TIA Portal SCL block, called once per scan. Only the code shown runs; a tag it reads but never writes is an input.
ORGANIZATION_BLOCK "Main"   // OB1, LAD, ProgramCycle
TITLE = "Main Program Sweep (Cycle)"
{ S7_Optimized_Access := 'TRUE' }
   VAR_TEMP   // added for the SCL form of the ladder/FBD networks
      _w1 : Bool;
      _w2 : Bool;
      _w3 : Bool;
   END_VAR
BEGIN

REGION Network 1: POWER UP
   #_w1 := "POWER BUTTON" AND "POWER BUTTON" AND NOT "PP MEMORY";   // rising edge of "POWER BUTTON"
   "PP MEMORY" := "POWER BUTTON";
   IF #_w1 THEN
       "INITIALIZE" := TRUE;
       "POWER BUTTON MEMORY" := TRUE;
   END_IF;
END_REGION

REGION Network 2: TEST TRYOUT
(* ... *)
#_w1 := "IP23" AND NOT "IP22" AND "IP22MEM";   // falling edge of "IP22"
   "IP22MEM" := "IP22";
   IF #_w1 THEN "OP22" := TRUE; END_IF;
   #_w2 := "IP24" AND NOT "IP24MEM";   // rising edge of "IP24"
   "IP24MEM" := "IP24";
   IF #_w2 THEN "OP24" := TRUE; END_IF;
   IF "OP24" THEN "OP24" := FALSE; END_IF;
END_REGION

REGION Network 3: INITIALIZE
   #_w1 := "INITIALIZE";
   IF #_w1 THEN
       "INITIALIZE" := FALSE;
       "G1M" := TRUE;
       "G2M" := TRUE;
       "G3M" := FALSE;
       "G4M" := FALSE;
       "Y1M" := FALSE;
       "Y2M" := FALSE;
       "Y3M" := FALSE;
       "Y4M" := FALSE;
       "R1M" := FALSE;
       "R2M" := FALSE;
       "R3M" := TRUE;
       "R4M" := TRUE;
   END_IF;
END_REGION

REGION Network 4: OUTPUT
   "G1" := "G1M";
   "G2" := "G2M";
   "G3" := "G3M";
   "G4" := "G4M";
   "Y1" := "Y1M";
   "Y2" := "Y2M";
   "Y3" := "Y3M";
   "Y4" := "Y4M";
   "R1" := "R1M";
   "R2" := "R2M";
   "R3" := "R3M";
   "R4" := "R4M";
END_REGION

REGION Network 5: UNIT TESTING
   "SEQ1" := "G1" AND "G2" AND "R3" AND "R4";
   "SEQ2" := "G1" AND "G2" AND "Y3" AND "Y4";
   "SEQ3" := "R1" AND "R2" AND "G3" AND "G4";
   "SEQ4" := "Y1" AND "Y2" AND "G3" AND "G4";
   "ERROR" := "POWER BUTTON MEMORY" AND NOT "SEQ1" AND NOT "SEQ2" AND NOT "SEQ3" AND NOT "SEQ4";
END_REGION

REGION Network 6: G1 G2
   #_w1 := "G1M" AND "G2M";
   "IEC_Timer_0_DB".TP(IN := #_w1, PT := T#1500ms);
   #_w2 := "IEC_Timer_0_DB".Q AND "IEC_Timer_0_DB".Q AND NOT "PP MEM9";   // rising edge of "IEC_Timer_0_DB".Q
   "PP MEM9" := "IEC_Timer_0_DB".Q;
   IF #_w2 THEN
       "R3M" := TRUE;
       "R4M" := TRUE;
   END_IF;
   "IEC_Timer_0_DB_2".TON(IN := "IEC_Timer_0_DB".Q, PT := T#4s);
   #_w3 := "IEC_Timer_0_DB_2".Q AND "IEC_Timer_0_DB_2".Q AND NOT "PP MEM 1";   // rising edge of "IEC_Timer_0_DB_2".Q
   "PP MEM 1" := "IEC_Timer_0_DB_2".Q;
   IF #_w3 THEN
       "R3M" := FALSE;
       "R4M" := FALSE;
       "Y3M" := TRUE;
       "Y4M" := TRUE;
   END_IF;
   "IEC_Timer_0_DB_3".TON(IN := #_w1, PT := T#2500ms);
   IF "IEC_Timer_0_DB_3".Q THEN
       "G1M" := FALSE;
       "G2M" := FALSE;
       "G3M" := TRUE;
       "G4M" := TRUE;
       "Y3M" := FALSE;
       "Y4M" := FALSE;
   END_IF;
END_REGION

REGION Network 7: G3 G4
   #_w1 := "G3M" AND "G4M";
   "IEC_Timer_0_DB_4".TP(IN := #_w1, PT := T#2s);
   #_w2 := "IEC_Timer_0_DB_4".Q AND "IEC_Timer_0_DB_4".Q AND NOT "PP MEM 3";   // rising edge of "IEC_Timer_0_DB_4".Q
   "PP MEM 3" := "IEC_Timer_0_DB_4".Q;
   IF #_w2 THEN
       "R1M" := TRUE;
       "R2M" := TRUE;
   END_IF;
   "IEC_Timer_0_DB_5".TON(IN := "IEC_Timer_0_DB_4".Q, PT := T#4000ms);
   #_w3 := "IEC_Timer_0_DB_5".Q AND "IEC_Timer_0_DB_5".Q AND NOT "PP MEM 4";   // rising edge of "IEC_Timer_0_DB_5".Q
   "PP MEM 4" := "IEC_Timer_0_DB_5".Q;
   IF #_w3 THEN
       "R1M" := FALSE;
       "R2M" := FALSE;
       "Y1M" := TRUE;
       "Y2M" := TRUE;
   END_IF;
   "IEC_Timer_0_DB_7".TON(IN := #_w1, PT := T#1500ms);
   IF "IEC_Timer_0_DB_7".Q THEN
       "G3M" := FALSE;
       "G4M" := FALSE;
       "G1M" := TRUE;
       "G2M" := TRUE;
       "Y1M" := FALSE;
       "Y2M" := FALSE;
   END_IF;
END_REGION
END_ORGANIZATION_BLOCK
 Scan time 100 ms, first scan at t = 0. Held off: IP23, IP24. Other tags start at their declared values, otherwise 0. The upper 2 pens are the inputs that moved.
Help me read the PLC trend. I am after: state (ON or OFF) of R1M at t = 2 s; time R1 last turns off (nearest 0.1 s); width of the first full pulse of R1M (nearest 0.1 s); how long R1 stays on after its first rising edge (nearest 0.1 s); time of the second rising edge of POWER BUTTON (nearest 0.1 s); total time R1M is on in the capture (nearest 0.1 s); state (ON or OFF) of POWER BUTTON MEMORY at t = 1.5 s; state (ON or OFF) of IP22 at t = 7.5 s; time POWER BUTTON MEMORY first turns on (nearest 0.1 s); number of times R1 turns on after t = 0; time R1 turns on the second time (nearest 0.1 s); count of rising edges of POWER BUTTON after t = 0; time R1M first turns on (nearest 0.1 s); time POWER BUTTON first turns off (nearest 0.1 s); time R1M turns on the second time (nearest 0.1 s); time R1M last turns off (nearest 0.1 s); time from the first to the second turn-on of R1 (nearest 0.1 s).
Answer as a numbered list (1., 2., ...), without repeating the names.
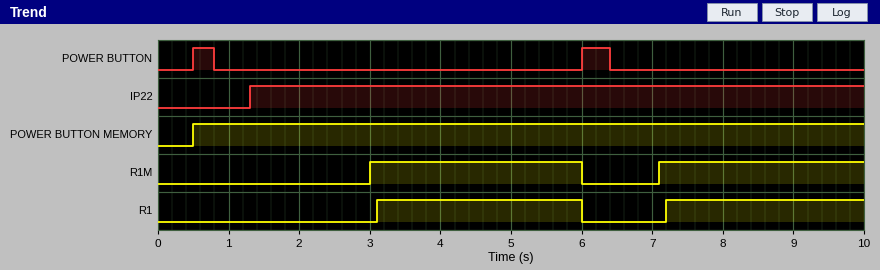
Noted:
1. OFF
2. 6.0 s
3. 3.0 s
4. 2.9 s
5. 6.0 s
6. 5.9 s
7. ON
8. ON
9. 0.5 s
10. 2
11. 7.2 s
12. 2
13. 3.0 s
14. 0.8 s
15. 7.1 s
16. 6.0 s
17. 4.1 s
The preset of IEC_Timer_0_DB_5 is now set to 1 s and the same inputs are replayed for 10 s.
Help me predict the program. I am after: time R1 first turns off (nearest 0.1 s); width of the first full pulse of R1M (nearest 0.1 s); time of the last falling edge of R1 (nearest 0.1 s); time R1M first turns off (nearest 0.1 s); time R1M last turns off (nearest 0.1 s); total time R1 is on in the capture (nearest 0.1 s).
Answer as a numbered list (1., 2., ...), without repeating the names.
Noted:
1. 4.1 s
2. 1.0 s
3. 8.2 s
4. 4.0 s
5. 8.1 s
6. 2.0 s
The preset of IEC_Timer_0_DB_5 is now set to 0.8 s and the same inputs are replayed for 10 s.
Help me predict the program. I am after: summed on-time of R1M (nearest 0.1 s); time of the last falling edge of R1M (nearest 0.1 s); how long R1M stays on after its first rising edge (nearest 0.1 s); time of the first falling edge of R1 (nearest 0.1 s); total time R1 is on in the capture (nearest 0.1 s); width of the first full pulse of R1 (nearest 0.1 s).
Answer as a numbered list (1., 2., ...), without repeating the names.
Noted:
1. 1.6 s
2. 7.9 s
3. 0.8 s
4. 3.9 s
5. 1.6 s
6. 0.8 s
